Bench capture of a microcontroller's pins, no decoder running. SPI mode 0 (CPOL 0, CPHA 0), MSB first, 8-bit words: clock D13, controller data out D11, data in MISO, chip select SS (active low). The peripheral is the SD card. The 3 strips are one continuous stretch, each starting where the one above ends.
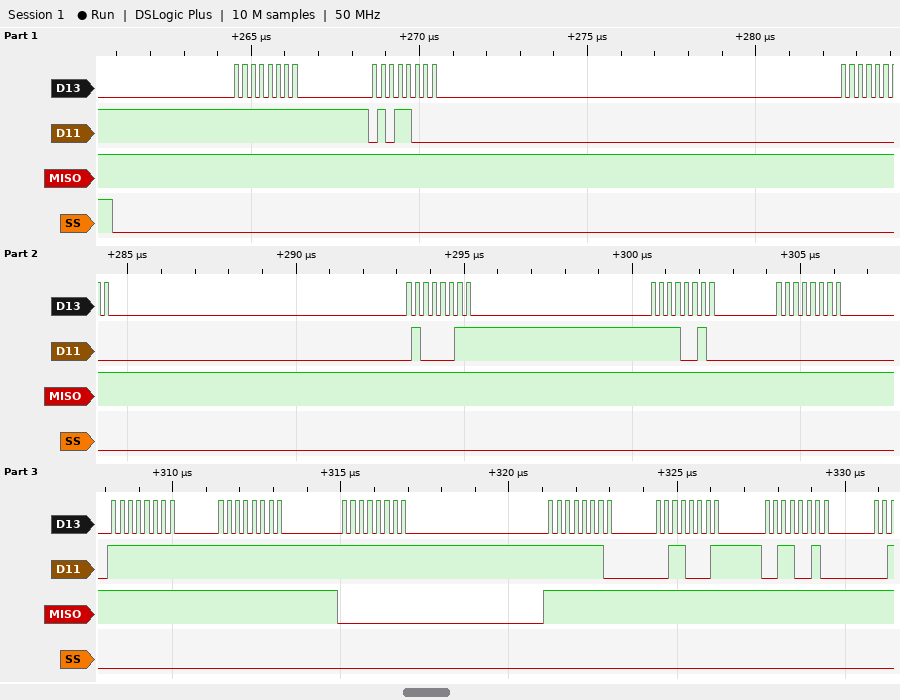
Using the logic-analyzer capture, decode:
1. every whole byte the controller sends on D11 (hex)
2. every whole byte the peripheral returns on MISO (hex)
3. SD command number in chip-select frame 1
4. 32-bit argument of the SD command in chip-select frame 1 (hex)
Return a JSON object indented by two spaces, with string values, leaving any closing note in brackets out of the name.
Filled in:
{
  "every whole byte the controller sends on D11": "0xFF 0x58 0x00 0x43 0xF2 0x00 0xFF 0xFF 0xFF 0xFE 0x31 0x32",
  "every whole byte the peripheral returns on MISO": "0xFF 0xFF 0xFF 0xFF 0xFF 0xFF 0xFF 0xFF 0x00 0xFF 0xFF 0xFF",
  "SD command number in chip-select frame 1": "CMD24",
  "32-bit argument of the SD command in chip-select frame 1": "0x0043F200"
}
